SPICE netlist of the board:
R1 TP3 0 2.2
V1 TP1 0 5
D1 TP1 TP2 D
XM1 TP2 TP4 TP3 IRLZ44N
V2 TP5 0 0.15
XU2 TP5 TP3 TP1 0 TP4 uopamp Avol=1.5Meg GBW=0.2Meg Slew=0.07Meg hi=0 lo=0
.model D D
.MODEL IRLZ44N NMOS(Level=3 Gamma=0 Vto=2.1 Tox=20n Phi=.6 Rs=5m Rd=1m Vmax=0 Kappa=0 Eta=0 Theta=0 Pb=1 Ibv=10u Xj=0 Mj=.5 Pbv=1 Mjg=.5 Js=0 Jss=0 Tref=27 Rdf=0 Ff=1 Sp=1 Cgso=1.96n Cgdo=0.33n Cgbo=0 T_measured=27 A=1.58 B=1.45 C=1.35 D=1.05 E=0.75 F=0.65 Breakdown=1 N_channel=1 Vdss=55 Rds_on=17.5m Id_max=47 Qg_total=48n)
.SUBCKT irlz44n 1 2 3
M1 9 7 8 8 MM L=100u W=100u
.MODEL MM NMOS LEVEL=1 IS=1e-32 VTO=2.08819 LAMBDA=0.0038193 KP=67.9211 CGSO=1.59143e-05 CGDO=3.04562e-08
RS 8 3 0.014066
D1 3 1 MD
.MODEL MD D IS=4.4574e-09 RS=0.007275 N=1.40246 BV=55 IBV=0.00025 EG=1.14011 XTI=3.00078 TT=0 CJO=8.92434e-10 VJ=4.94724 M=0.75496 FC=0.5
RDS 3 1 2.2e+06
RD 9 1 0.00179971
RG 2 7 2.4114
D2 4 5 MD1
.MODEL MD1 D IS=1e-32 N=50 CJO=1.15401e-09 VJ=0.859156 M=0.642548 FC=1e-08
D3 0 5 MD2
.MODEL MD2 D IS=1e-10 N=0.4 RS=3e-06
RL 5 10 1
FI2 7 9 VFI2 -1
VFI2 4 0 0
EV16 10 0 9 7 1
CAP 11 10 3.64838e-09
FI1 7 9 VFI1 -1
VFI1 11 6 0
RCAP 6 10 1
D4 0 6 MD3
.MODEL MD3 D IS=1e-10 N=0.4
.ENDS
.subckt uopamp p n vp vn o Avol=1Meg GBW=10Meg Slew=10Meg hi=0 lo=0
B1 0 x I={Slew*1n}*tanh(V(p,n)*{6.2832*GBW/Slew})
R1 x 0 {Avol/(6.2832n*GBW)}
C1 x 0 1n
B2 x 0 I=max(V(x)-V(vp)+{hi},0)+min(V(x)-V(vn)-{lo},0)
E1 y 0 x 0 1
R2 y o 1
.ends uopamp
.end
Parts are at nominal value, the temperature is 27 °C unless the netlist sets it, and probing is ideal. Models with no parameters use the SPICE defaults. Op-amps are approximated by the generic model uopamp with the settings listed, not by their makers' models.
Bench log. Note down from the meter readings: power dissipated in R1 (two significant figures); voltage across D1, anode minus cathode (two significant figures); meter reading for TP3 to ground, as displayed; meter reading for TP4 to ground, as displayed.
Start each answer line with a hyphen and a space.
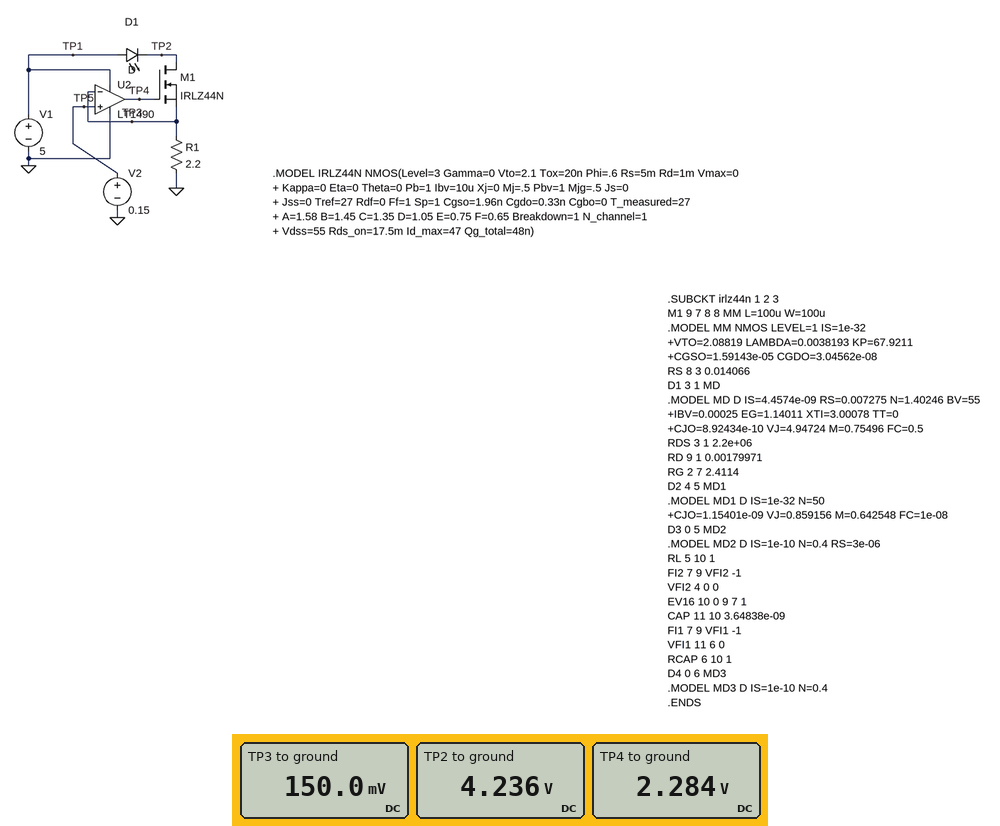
- 10 mW
- 760 mV
- 150.0 mV
- 2.284 V
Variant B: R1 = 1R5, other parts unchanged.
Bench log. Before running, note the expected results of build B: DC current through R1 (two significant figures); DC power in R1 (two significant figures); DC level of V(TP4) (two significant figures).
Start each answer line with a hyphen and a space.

- 100 mA
- 15 mW
- 2.3 V
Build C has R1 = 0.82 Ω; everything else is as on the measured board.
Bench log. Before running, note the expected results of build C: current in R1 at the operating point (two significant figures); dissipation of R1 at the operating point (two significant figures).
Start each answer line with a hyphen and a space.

- 180 mA
- 27 mW
